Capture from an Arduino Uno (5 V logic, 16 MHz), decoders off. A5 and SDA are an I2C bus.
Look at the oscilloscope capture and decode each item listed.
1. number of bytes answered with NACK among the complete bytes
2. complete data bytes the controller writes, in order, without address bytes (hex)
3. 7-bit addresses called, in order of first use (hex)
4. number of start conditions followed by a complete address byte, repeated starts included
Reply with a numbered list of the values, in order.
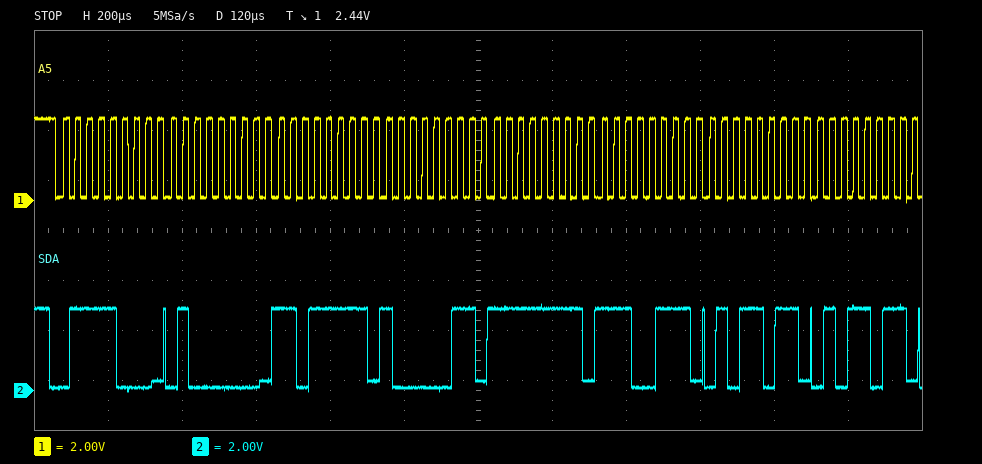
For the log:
1. 0
2. 40 DF 83 FF E7 5B 5B
3. 0x3C
4. 1
